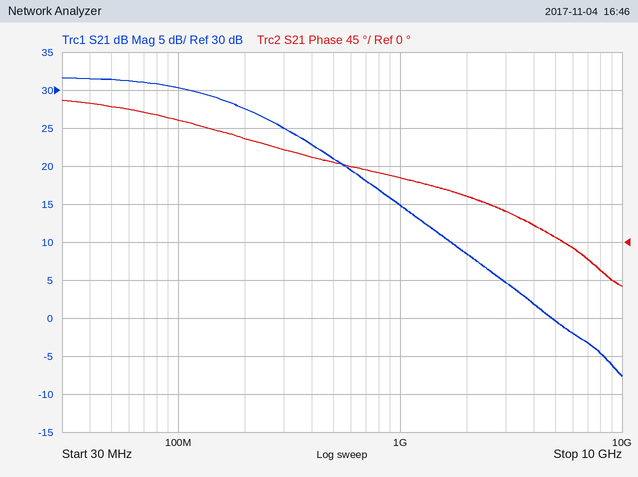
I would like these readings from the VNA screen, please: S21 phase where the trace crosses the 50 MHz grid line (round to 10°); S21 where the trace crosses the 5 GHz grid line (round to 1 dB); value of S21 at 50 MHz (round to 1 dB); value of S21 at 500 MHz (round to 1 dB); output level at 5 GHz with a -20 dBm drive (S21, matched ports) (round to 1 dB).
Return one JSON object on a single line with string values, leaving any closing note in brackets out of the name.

{"S21 phase where the trace crosses the 50 MHz grid line": "160°", "S21 where the trace crosses the 5 GHz grid line": "0 dB", "value of S21 at 50 MHz": "31 dB", "value of S21 at 500 MHz": "21 dB", "output level at 5 GHz with a -20 dBm drive (S21, matched ports)": "-20 dBm"}
